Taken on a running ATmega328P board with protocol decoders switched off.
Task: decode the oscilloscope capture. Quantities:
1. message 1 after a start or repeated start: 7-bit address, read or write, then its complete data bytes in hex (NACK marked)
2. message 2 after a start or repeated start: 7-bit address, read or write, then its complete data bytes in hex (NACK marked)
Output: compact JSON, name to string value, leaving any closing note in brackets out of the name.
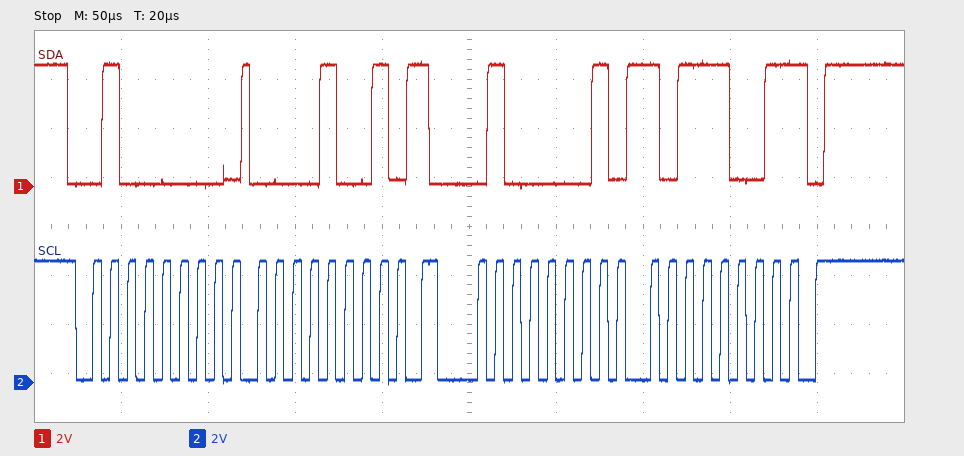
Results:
{"message 1 after a start or repeated start: 7-bit address, read or write, then its complete data bytes in hex": "0x20 write: 09", "message 2 after a start or repeated start: 7-bit address, read or write, then its complete data bytes in hex": "0x20 read: B9 NACK"}
